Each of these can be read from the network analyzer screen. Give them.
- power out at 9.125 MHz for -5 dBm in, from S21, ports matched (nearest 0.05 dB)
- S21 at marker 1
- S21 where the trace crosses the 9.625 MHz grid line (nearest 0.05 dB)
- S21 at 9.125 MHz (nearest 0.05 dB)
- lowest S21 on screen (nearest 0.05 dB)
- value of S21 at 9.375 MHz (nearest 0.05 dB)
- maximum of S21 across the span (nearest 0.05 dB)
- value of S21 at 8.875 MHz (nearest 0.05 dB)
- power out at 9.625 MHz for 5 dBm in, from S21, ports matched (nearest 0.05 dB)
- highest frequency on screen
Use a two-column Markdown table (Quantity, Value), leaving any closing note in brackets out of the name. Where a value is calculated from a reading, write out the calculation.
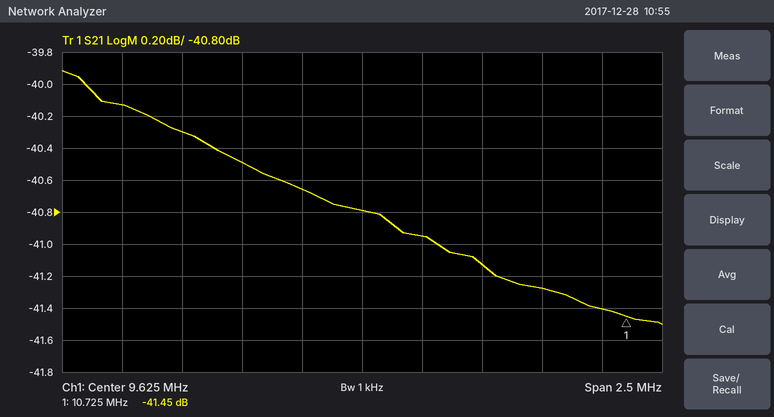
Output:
| Quantity | Value |
|---|---|
| power out at 9.125 MHz for -5 dBm in, from S21, ports matched | -5 dBm + (-40.50 dB) = -45.50 dBm |
| S21 at marker 1 | -41.45 dB |
| S21 where the trace crosses the 9.625 MHz grid line | -40.80 dB |
| S21 at 9.125 MHz | -40.50 dB |
| lowest S21 on screen | -41.50 dB |
| value of S21 at 9.375 MHz | -40.65 dB |
| maximum of S21 across the span | -39.90 dB |
| value of S21 at 8.875 MHz | -40.30 dB |
| power out at 9.625 MHz for 5 dBm in, from S21, ports matched | 5 dBm + (-40.80 dB) = -35.80 dBm |
| highest frequency on screen | 10.875 MHz |
